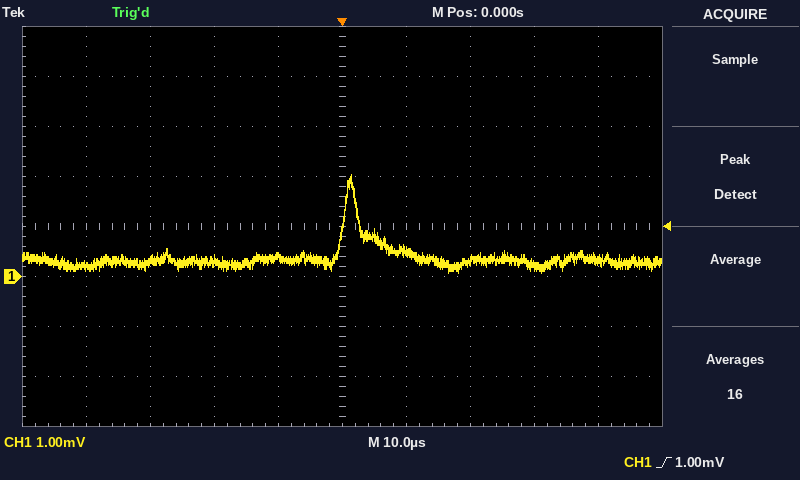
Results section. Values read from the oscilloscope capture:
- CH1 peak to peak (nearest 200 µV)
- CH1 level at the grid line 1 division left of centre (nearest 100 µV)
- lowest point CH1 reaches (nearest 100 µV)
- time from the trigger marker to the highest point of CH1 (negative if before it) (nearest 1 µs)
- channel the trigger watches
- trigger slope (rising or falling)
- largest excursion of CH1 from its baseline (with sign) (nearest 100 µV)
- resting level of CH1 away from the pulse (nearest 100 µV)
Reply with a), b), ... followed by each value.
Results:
a) 2.0 mV
b) 400 µV
c) 100 µV
d) +1 µs
e) CH1
f) rising
g) +1.7 mV
h) 300 µV
